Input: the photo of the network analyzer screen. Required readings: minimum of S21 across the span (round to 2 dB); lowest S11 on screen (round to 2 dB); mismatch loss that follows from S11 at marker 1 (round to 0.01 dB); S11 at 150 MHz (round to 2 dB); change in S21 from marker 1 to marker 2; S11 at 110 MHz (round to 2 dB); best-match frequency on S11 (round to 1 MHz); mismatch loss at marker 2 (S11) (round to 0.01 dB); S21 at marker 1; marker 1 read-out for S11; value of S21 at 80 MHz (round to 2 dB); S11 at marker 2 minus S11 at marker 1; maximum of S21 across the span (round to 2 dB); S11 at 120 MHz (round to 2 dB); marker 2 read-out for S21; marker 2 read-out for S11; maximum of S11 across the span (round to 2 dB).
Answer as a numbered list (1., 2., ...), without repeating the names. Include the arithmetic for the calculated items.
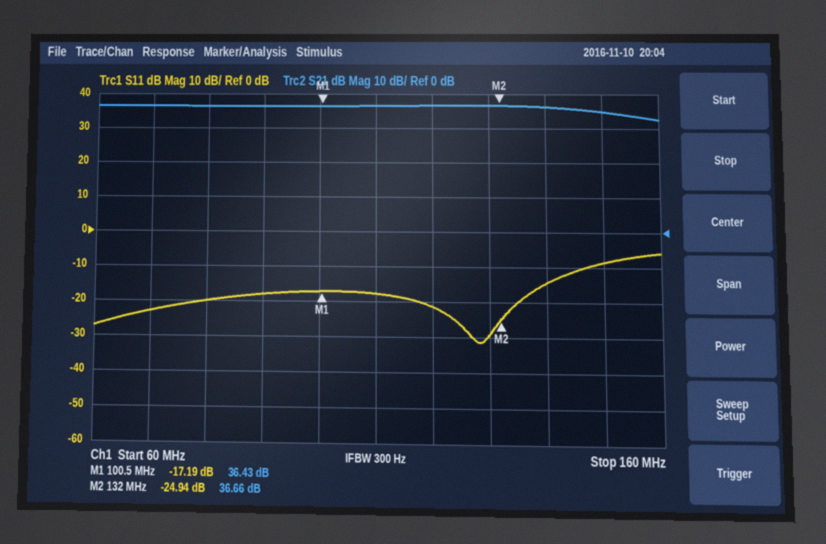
1. 32 dB
2. -32 dB
3. −10 log10(1 − 10^(-17.19/10)) ≈ 0.08 dB
4. -8 dB
5. 36.66 − (36.43) = 0.23 dB
6. -18 dB
7. 128 MHz
8. −10 log10(1 − 10^(-24.94/10)) ≈ 0.01 dB
9. 36.43 dB
10. -17.19 dB
11. 36 dB
12. -24.94 − (-17.19) = -7.75 dB
13. 36 dB
14. -22 dB
15. 36.66 dB
16. -24.94 dB
17. -6 dB
